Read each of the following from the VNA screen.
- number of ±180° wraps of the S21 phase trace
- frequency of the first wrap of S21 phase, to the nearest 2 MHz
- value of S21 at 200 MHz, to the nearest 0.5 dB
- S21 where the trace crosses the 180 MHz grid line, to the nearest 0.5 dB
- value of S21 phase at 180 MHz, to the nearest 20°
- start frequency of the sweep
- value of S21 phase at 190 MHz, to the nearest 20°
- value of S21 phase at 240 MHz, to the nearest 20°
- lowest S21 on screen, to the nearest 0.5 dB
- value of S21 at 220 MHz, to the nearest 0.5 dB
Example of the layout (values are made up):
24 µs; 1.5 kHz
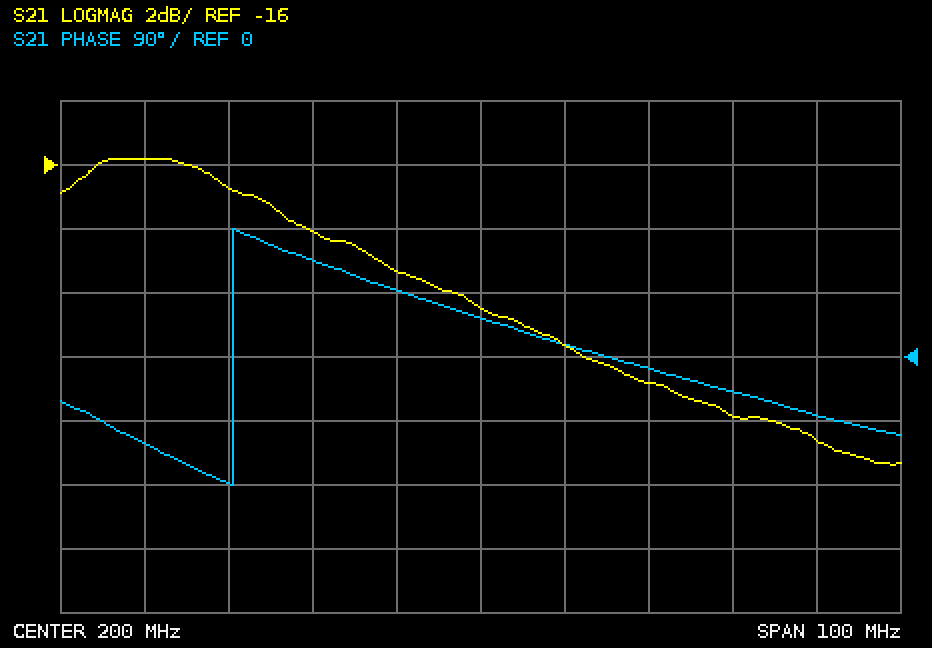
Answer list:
1; 170 MHz; -20.5 dB; -18.0 dB; 140°; 150 MHz; 100°; -80°; -25.5 dB; -23.0 dB
